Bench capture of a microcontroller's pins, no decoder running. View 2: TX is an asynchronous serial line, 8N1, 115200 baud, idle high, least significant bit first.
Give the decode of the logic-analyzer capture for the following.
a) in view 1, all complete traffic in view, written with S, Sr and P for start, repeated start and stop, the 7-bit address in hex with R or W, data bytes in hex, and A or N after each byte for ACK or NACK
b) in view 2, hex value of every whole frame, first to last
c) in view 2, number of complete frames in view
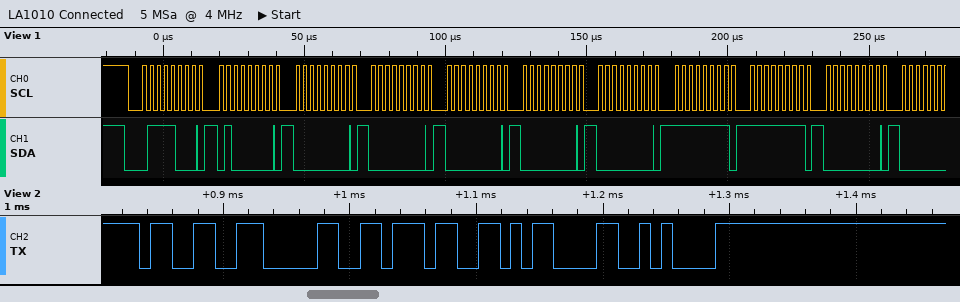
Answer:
S 3CW A 40 A 00 A 00 A 00 A 00 A 00 A FF A FF A 00 A
33 30 37 0D 0A
5
